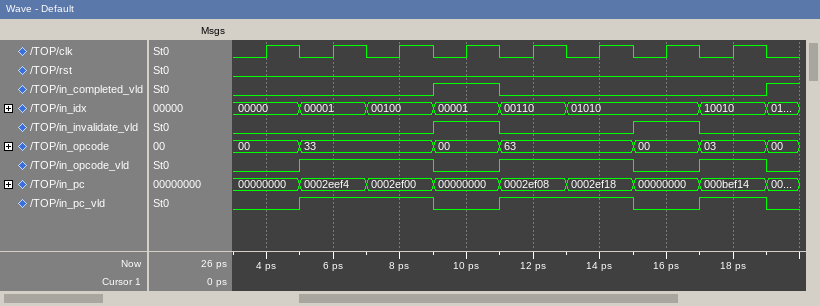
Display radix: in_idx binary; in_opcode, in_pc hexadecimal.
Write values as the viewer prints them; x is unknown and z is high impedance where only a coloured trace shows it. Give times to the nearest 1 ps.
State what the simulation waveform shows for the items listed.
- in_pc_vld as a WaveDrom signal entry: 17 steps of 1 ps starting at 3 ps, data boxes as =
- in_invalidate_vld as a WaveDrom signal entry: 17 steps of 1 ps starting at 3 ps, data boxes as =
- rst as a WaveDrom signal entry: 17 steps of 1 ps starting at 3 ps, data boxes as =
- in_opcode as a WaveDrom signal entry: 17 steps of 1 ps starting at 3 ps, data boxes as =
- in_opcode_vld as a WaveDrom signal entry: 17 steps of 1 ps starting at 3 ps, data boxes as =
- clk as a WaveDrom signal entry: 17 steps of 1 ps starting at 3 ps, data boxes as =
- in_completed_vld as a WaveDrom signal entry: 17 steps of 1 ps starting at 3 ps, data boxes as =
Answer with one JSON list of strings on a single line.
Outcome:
["{name: 'in_pc_vld', wave: '0.1...0.1...0.1.0'}", "{name: 'in_invalidate_vld', wave: '0.....1.0...1.0..'}", "{name: 'rst', wave: '0................'}", "{name: 'in_opcode', wave: '=.=...=.=...=.=.=', data: '00 33 00 63 00 03 00'}", "{name: 'in_opcode_vld', wave: '0.1...0.1...0.1.0'}", "{name: 'clk', wave: '01010101010101010'}", "{name: 'in_completed_vld', wave: '0.....1.0.......1'}"]
